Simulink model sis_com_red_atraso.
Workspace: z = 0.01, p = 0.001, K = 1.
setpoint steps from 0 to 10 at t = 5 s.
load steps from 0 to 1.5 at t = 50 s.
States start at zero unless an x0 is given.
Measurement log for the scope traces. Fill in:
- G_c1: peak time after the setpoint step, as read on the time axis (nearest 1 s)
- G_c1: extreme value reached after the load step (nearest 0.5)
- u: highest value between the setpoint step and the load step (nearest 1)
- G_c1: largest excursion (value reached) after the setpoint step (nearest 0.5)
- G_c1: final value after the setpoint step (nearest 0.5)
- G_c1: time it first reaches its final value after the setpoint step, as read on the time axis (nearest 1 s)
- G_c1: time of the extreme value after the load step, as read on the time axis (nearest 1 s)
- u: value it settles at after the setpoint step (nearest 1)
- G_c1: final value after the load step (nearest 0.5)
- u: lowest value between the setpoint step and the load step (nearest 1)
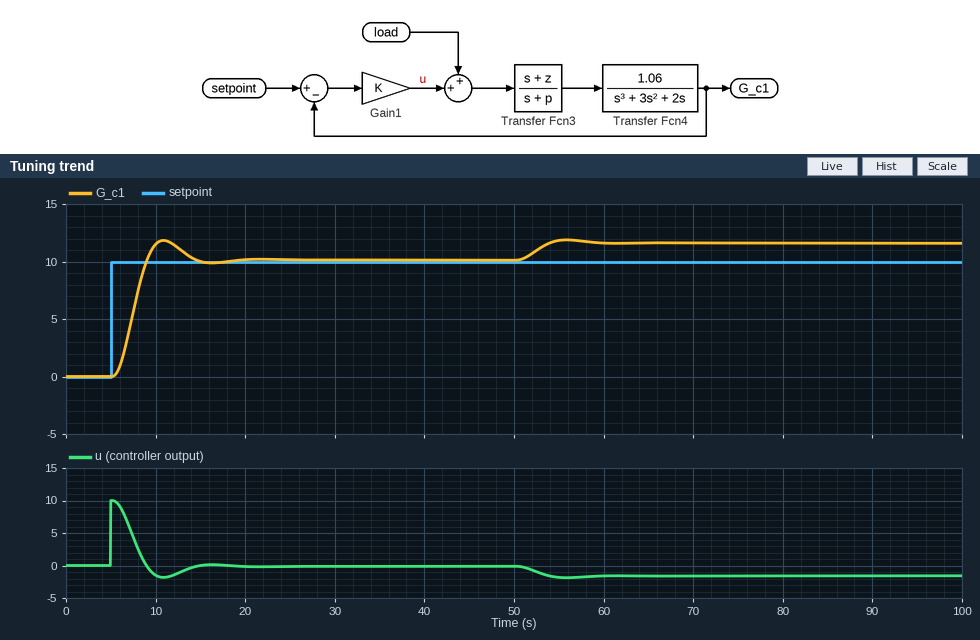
11 s
12.0
10
12.0
10.0
9 s
56 s
0
11.5
-2
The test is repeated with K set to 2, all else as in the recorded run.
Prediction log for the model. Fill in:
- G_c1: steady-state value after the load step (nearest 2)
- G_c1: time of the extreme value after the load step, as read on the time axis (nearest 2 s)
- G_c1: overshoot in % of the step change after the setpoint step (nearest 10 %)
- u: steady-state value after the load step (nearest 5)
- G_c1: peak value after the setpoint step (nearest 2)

10
54 s
40 %
0
14
